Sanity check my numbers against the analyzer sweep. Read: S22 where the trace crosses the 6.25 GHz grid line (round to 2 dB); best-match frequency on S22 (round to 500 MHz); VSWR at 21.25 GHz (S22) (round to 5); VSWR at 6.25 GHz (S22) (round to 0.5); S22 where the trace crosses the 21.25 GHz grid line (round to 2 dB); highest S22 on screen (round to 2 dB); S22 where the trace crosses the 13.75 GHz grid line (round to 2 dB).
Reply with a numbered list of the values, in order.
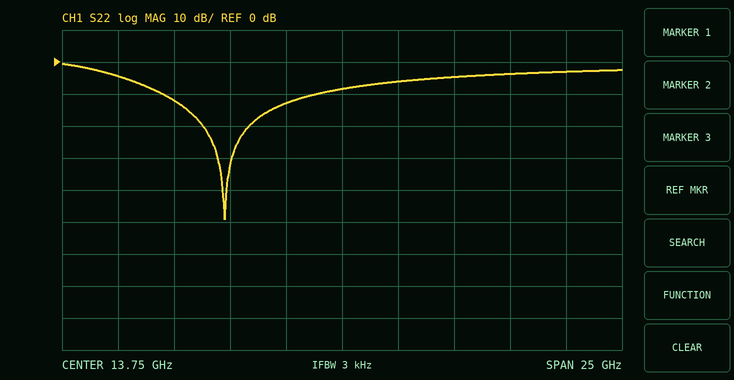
1. -12 dB
2. 8.5 GHz
3. 5
4. 1.5
5. -4 dB
6. 0 dB
7. -8 dB
